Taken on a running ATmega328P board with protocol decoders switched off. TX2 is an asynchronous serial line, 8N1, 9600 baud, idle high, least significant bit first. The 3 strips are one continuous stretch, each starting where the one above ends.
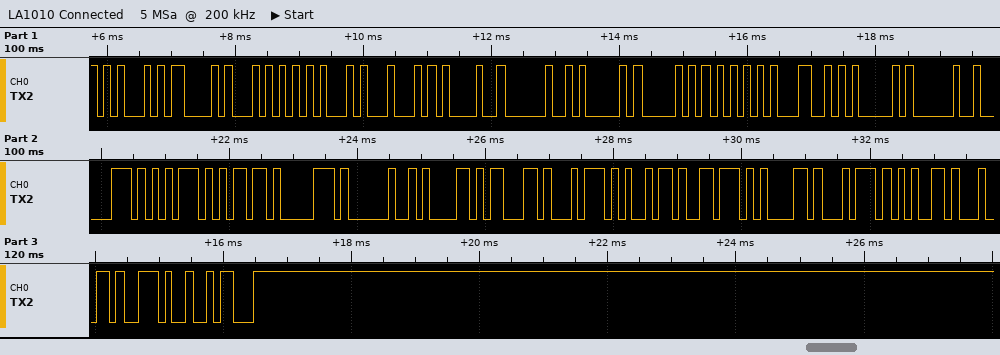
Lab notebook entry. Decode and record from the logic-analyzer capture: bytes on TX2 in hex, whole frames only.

45 43 54 45 44 21 20 41 50 55 4C 41 20 70 75 6D 70 20 61 63 74 69 76 61 74 65 64 2E 1A
